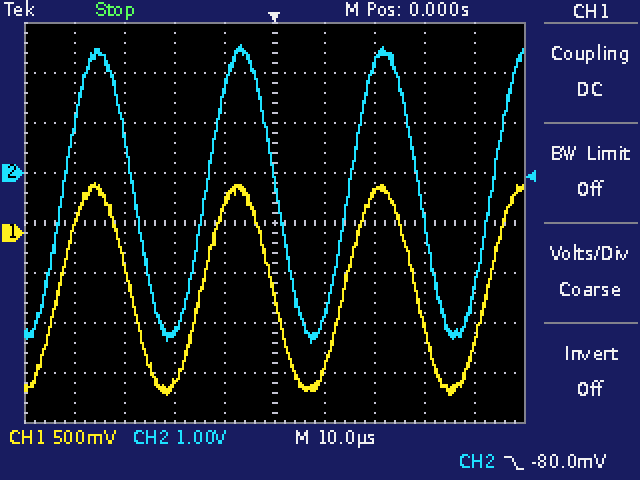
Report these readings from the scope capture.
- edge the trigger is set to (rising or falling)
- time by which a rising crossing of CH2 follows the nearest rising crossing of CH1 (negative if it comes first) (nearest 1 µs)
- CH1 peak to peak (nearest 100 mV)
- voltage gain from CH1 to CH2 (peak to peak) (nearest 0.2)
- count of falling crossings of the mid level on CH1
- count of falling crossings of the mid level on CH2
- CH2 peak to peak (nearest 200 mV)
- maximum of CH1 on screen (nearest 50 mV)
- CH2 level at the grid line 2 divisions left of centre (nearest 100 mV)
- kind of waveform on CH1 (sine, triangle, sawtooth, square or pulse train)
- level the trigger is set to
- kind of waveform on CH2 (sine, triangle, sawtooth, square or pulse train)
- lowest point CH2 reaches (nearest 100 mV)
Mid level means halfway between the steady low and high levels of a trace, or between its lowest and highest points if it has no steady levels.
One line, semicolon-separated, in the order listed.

falling; +1 µs; 2.10 V; 2.8; 3; 3; 6.0 V; 500 mV; -3.2 V; sine; -80.0 mV; sine; -3.4 V
